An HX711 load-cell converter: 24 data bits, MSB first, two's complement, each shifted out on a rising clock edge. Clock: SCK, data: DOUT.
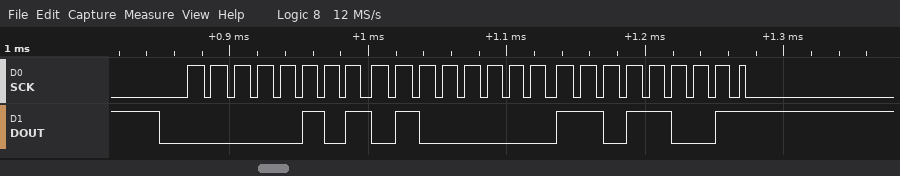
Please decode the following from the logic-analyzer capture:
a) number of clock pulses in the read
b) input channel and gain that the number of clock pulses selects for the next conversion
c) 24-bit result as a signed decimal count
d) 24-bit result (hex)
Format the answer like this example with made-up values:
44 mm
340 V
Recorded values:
25
channel A, gain 128
344281
0x0540D9
